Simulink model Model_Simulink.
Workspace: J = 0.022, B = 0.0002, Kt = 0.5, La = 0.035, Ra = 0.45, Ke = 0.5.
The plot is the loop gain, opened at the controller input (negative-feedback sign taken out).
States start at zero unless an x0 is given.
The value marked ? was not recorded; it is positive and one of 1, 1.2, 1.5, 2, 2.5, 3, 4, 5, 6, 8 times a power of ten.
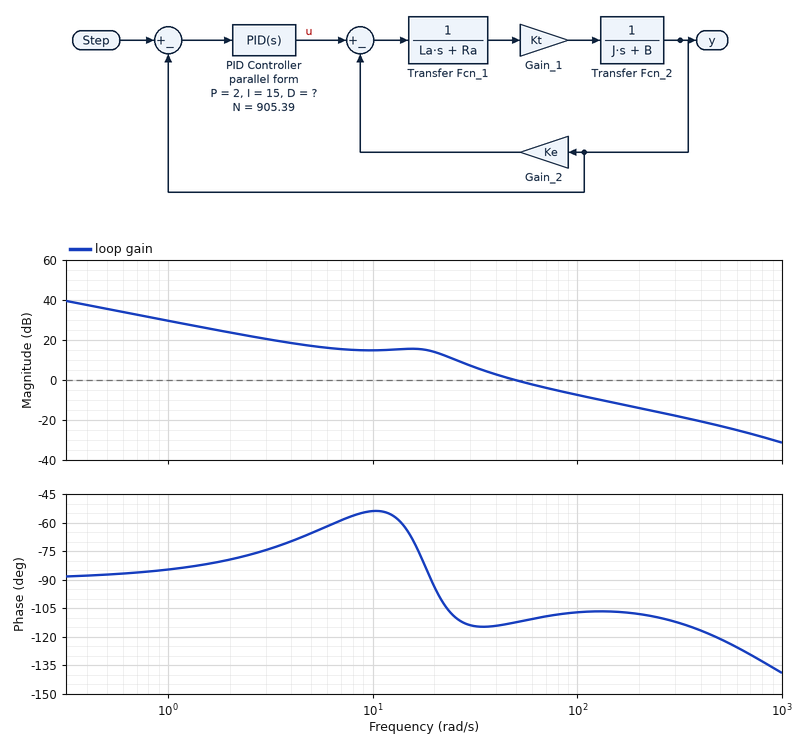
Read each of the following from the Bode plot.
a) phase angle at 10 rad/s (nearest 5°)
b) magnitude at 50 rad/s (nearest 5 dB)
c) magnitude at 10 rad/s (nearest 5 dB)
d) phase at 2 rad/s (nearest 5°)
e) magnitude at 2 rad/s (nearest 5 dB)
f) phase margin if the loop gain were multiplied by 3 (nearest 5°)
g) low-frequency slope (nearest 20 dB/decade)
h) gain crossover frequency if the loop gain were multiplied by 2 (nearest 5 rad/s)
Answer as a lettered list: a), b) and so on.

a) -55°
b) 0 dB
c) 15 dB
d) -80°
e) 25 dB
f) 75°
g) -20 dB/decade
h) 85 rad/s
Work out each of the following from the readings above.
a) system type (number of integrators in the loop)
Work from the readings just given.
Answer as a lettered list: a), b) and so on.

a) 1
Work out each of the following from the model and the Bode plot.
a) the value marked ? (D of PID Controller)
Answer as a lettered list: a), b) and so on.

a) 0.06
